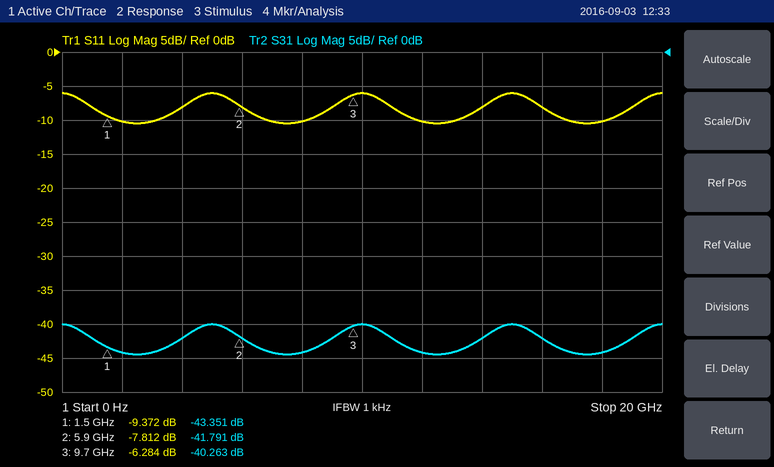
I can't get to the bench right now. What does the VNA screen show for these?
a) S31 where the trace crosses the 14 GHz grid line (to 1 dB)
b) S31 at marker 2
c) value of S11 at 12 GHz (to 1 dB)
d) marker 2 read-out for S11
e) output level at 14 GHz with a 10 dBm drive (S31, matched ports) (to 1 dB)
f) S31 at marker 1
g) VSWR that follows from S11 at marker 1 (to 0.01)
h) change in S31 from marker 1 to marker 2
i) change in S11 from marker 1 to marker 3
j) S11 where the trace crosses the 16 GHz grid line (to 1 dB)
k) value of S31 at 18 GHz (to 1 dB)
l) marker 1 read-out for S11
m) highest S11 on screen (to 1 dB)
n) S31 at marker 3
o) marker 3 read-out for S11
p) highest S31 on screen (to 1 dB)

-42 dB
-41.791 dB
-10 dB
-7.812 dB
-32 dBm
-43.351 dB
2.03
1.560 dB
3.088 dB
-8 dB
-44 dB
-9.372 dB
-6 dB
-40.263 dB
-6.284 dB
-40 dB
